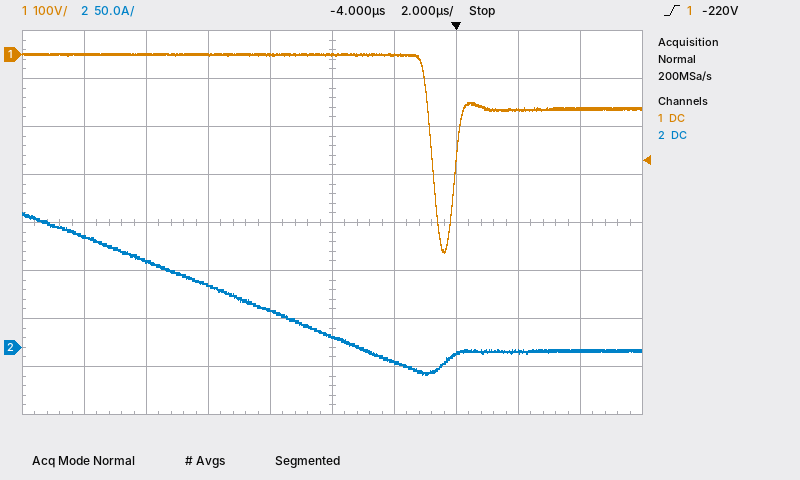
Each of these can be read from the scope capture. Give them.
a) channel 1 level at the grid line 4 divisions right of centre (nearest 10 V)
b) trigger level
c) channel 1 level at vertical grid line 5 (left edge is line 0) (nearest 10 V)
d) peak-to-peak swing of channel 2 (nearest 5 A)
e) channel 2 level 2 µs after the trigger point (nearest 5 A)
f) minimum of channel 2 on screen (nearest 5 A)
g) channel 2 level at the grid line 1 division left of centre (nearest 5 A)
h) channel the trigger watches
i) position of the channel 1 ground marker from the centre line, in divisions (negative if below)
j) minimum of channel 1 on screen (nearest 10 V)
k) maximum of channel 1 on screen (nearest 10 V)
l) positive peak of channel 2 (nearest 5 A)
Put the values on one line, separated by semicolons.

-110 V; -220 V; 0 V; 170 A; -5 A; -30 A; 40 A; channel 1; +3.5 div; -410 V; 0 V; 140 A
